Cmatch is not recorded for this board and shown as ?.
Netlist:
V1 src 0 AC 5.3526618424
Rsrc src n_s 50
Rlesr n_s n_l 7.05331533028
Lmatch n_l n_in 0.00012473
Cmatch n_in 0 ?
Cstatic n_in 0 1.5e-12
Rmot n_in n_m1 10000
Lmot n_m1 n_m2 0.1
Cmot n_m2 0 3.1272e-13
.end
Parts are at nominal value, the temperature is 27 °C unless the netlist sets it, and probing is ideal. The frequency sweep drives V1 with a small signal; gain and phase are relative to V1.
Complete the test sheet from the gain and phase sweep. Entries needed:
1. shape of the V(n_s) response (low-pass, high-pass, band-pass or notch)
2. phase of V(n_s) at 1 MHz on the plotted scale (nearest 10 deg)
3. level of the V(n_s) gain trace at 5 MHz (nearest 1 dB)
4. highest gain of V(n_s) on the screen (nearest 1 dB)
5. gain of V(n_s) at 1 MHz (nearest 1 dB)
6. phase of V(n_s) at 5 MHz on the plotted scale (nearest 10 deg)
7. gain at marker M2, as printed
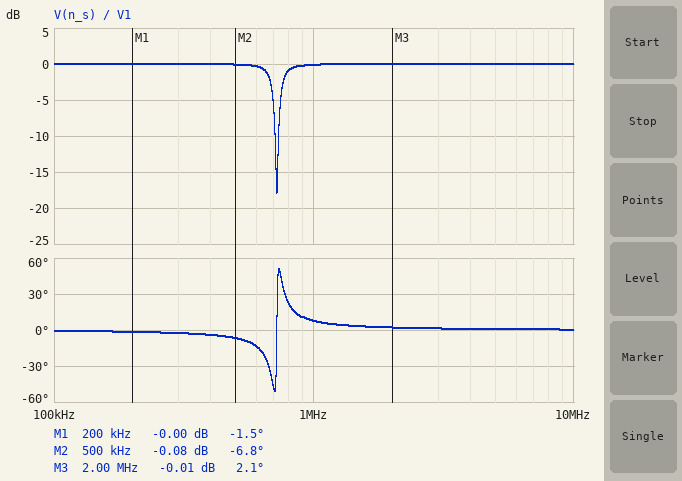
notch
10 deg
0 dB
0 dB
0 dB
0 deg
-0.08 dB
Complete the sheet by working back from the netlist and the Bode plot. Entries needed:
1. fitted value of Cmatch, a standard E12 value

390 pF
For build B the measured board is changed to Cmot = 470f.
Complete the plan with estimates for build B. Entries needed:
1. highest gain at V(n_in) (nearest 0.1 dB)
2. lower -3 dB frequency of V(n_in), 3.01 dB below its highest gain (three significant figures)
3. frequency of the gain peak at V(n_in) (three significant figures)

19.4 dB
674 kHz
708 kHz
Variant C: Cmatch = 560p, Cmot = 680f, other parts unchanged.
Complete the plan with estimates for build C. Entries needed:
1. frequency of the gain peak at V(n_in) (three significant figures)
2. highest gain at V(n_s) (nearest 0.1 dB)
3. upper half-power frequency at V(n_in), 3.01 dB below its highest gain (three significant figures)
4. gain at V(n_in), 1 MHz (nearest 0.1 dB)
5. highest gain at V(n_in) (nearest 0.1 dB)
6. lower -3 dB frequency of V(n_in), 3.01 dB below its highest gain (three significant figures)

589 kHz
0 dB
642 kHz
-5.0 dB
17.8 dB
555 kHz
